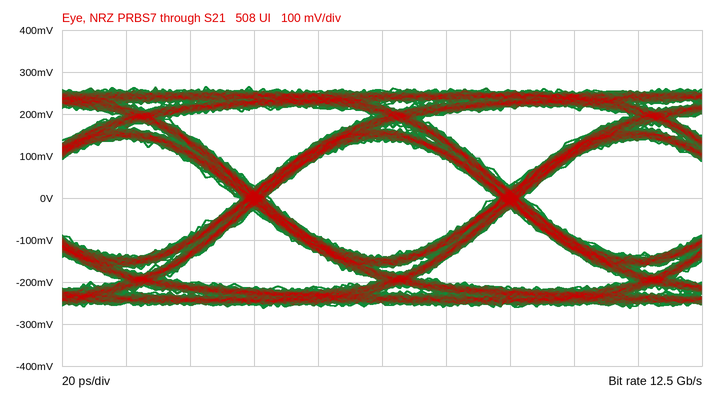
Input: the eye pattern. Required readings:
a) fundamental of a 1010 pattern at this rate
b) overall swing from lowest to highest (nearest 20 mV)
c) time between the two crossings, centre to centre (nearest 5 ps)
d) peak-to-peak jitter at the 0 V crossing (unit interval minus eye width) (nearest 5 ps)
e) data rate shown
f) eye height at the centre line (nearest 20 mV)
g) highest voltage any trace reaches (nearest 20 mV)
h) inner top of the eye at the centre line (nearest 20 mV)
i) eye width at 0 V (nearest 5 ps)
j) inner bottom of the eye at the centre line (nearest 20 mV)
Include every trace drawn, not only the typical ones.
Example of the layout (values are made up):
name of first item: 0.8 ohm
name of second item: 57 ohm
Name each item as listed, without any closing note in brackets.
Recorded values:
fundamental of a 1010 pattern at this rate: 6.25 GHz
overall swing from lowest to highest: 520 mV
time between the two crossings, centre to centre: 80 ps
peak-to-peak jitter at the 0 V crossing (unit interval minus eye width): 10 ps
data rate shown: 12.5 Gb/s
eye height at the centre line: 280 mV
highest voltage any trace reaches: 260 mV
inner top of the eye at the centre line: 140 mV
eye width at 0 V: 70 ps
inner bottom of the eye at the centre line: -140 mV
